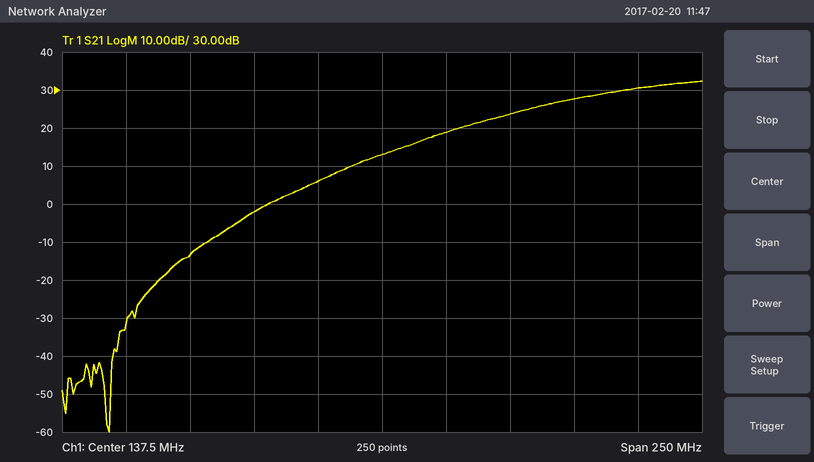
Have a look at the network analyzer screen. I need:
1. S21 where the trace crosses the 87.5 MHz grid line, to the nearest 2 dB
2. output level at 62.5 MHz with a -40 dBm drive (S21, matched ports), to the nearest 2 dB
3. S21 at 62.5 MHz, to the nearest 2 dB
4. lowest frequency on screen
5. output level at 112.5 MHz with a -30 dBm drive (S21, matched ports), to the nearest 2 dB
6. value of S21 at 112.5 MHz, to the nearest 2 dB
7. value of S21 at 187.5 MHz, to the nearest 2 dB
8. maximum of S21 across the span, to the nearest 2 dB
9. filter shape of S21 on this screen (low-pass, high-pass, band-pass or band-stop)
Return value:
-2 dB
-54 dBm
-14 dB
12.5 MHz
-24 dBm
6 dB
24 dB
32 dB
high-pass
